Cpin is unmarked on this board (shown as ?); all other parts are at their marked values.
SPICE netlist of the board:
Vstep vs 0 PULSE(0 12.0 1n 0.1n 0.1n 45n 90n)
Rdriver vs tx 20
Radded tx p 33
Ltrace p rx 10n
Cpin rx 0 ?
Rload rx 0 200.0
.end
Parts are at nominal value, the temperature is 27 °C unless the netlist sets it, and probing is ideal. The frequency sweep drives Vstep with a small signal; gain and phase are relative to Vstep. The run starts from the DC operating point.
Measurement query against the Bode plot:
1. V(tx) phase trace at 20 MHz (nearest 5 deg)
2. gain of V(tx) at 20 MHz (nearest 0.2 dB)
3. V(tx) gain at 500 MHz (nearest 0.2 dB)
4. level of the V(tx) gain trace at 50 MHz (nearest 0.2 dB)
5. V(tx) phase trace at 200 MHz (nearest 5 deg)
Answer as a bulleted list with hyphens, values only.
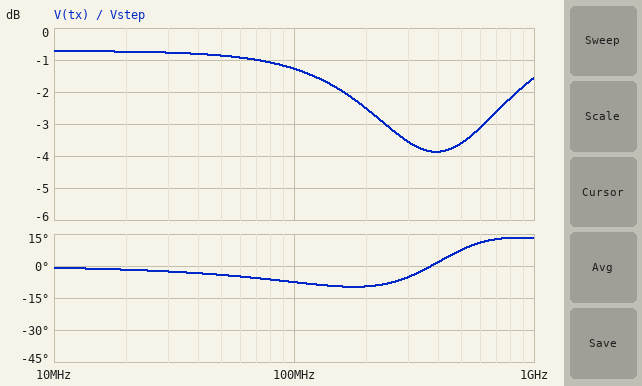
- 0 deg
- -0.8 dB
- -3.6 dB
- -0.8 dB
- -10 deg
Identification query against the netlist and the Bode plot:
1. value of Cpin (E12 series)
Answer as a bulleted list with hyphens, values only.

- 18 pF
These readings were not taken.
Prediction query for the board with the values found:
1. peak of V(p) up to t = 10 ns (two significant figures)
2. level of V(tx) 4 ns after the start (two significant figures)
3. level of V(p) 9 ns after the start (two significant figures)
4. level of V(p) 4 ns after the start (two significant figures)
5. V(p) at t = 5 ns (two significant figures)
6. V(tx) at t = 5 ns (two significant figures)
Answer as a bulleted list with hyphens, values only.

- 9.5 V
- 11 V
- 9.5 V
- 9.4 V
- 9.5 V
- 11 V
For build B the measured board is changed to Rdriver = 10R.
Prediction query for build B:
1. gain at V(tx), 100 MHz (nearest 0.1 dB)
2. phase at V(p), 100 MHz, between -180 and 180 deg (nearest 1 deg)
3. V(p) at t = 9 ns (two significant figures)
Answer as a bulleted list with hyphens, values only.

- -0.6 dB
- -22 deg
- 9.9 V
